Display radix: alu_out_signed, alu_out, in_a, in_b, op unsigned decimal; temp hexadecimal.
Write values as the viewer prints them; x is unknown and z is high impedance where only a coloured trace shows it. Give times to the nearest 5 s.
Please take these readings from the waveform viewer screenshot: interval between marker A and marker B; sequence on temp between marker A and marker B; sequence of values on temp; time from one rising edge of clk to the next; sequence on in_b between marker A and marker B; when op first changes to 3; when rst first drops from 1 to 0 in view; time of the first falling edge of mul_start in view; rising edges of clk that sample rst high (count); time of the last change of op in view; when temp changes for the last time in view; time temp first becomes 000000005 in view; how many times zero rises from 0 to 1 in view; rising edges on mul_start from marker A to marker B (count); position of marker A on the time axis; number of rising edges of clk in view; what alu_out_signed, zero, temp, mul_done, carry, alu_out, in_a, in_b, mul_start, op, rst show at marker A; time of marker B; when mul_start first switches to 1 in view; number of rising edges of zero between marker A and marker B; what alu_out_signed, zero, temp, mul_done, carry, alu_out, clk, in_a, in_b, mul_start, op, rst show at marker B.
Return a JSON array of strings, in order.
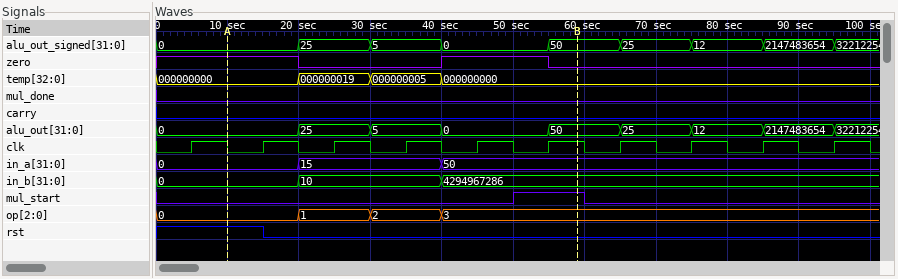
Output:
["50 s", "000000000, 000000019, 000000005, 000000000", "000000000, 000000019, 000000005, 000000000", "10 s", "0, 10, 4294967286", "40 s", "15 s", "60 s", "2", "40 s", "40 s", "30 s", "1", "1", "10 s", "10", "alu_out_signed=0, zero=1, temp=000000000, mul_done=0, carry=0, alu_out=0, in_a=0, in_b=0, mul_start=0, op=0, rst=1", "60 s", "50 s", "1", "alu_out_signed=50, zero=0, temp=000000000, mul_done=0, carry=0, alu_out=50, clk=1, in_a=50, in_b=4294967286, mul_start=1, op=3, rst=0"]
